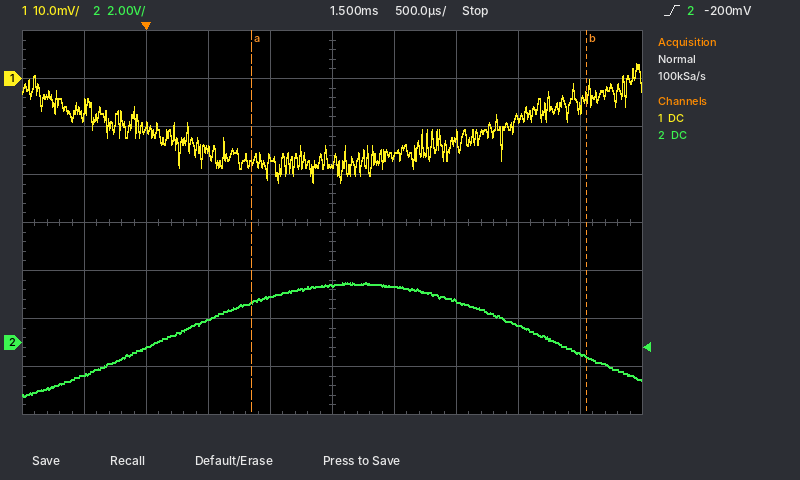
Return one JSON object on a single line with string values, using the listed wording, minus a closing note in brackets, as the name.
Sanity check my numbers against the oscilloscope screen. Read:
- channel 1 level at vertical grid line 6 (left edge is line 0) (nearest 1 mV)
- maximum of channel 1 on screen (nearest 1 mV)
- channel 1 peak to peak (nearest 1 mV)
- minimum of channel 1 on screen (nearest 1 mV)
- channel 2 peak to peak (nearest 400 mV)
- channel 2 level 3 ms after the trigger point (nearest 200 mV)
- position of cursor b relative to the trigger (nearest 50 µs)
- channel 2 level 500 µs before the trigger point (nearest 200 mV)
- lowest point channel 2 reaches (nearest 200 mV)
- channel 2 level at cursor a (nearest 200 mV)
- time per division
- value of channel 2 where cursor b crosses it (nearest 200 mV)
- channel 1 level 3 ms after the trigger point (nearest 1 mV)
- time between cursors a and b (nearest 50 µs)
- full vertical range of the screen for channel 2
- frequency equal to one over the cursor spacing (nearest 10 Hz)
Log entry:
{"channel 1 level at vertical grid line 6 (left edge is line 0)": "-16 mV", "maximum of channel 1 on screen": "3 mV", "channel 1 peak to peak": "25 mV", "minimum of channel 1 on screen": "-22 mV", "channel 2 peak to peak": "4.8 V", "channel 2 level 3 ms after the trigger point": "800 mV", "position of cursor b relative to the trigger": "+3.55 ms", "channel 2 level 500 µs before the trigger point": "-1.4 V", "lowest point channel 2 reaches": "-2.2 V", "channel 2 level at cursor a": "1.6 V", "time per division": "500 µs", "value of channel 2 where cursor b crosses it": "-600 mV", "channel 1 level 3 ms after the trigger point": "-8 mV", "time between cursors a and b": "2.70 ms", "full vertical range of the screen for channel 2": "16 V", "frequency equal to one over the cursor spacing": "370 Hz"}
